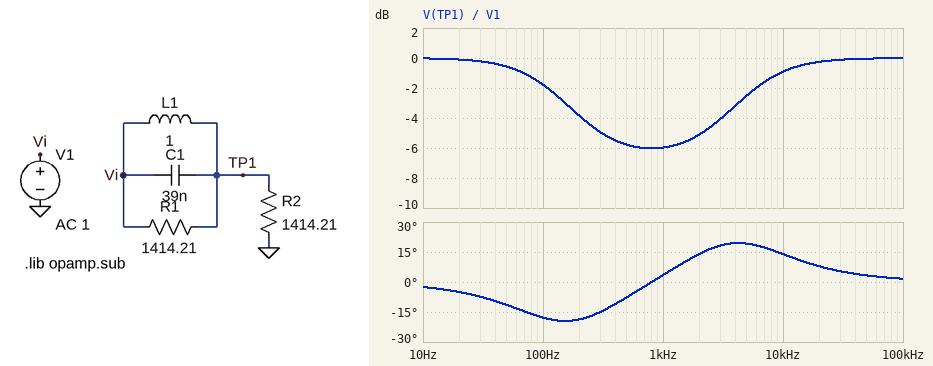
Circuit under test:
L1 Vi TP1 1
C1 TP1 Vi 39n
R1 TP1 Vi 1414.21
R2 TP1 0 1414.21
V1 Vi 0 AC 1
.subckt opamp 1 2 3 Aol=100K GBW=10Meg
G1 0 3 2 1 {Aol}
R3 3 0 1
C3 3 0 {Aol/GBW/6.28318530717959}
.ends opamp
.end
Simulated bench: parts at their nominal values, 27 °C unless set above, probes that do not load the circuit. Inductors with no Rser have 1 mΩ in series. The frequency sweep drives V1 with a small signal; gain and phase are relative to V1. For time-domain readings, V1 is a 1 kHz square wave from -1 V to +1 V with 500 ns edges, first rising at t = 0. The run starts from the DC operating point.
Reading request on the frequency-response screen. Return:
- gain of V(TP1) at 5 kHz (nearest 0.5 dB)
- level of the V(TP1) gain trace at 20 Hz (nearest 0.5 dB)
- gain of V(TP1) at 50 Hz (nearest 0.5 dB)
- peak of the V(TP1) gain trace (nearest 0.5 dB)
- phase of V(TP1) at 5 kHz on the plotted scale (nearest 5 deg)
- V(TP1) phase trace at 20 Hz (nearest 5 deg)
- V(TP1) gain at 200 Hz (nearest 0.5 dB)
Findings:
-2.5 dB
0 dB
-0.5 dB
0 dB
20 deg
-5 deg
-4.0 dB
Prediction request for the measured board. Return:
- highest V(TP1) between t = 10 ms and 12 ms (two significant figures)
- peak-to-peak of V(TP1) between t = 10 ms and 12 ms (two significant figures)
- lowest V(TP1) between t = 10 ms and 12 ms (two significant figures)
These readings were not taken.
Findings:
1.4 V
2.8 V
-1.4 V
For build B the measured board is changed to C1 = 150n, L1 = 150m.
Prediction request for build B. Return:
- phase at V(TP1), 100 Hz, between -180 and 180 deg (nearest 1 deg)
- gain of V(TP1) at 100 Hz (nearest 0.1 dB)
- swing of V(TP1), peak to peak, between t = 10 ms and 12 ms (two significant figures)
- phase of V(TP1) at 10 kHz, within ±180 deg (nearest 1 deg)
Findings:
-4 deg
-0.1 dB
2.3 V
4 deg
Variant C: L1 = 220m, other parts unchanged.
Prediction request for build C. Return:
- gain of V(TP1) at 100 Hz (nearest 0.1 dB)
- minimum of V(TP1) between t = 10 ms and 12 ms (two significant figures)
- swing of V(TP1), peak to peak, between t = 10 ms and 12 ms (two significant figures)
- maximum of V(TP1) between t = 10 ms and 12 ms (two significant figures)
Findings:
-0.1 dB
-1.2 V
2.3 V
1.2 V
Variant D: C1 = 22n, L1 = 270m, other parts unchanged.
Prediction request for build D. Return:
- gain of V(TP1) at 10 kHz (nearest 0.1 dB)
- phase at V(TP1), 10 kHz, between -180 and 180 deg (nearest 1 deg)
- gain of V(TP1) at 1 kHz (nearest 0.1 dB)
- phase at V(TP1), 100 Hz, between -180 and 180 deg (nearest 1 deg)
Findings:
-2.2 dB
19 deg
-5.0 dB
-7 deg
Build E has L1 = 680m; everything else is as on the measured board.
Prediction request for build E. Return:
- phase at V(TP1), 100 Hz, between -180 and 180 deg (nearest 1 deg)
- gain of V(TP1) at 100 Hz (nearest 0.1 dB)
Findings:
-14 deg
-1.0 dB
